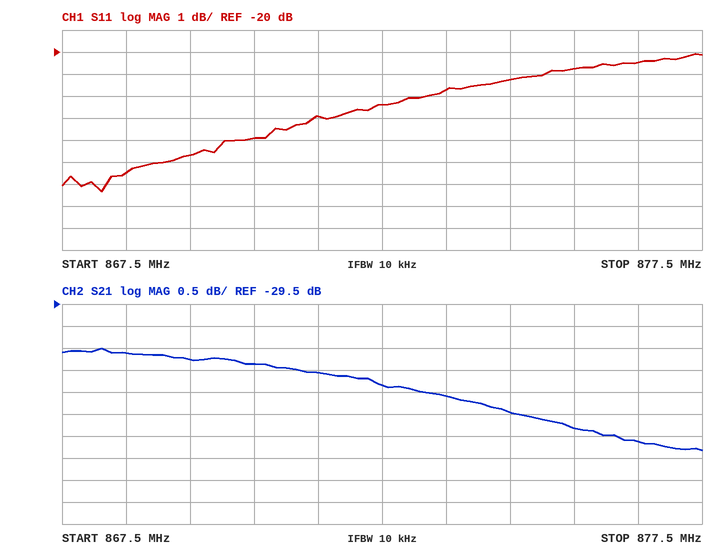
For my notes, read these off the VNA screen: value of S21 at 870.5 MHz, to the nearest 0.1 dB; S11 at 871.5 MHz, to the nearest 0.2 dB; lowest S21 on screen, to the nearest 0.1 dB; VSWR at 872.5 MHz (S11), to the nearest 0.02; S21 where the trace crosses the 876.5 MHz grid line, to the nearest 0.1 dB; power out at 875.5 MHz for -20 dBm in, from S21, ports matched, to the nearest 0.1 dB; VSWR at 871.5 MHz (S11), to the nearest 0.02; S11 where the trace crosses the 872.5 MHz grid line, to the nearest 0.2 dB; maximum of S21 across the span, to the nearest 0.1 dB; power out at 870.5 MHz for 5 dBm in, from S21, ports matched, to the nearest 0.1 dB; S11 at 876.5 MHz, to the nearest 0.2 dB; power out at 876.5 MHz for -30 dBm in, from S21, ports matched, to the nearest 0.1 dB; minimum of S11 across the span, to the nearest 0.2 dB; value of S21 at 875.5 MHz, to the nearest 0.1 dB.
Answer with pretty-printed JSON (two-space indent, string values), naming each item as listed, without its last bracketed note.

{
  "value of S21 at 870.5 MHz, to the nearest 0.1 dB": "-30.9 dB",
  "S11 at 871.5 MHz, to the nearest 0.2 dB": "-23.0 dB",
  "lowest S21 on screen, to the nearest 0.1 dB": "-32.8 dB",
  "VSWR at 872.5 MHz (S11), to the nearest 0.02": "1.16",
  "S21 where the trace crosses the 876.5 MHz grid line, to the nearest 0.1 dB": "-32.6 dB",
  "power out at 875.5 MHz for -20 dBm in, from S21, ports matched, to the nearest 0.1 dB": "-52.3 dBm",
  "VSWR at 871.5 MHz (S11), to the nearest 0.02": "1.16",
  "S11 where the trace crosses the 872.5 MHz grid line, to the nearest 0.2 dB": "-22.4 dB",
  "maximum of S21 across the span, to the nearest 0.1 dB": "-30.5 dB",
  "power out at 870.5 MHz for 5 dBm in, from S21, ports matched, to the nearest 0.1 dB": "-25.9 dBm",
  "S11 at 876.5 MHz, to the nearest 0.2 dB": "-20.4 dB",
  "power out at 876.5 MHz for -30 dBm in, from S21, ports matched, to the nearest 0.1 dB": "-62.6 dBm",
  "minimum of S11 across the span, to the nearest 0.2 dB": "-26.4 dB",
  "value of S21 at 875.5 MHz, to the nearest 0.1 dB": "-32.3 dB"
}
